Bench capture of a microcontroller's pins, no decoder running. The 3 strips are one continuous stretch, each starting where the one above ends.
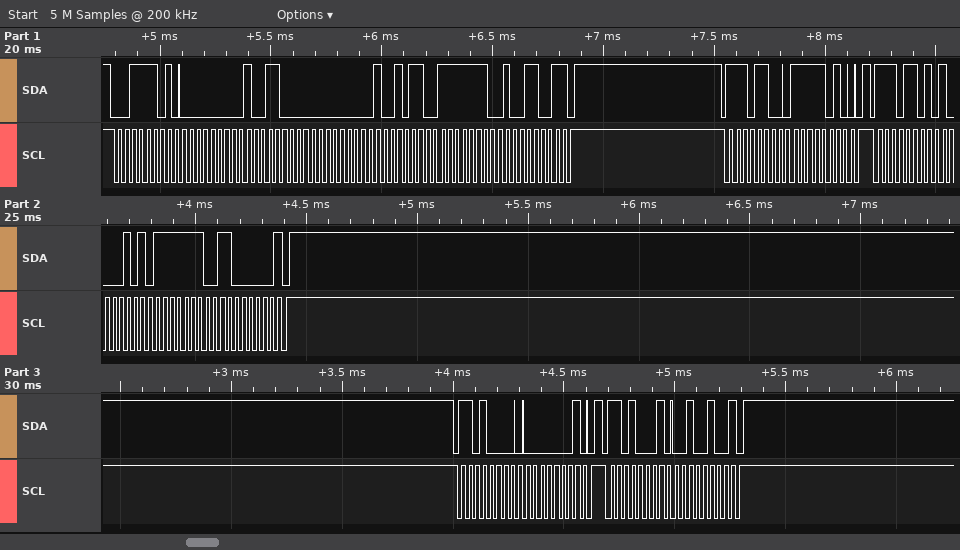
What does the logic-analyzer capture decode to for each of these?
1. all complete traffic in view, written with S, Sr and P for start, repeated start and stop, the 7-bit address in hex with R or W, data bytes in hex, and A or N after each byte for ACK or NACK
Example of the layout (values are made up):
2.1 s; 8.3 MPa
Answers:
S 1ER A 00 A 98 A 00 A 96 A FE A 99 N P S 76W A FA A P S 76R A 85 A FE A C0 N P S 68W A 01 A P S 68R A 24 N P
